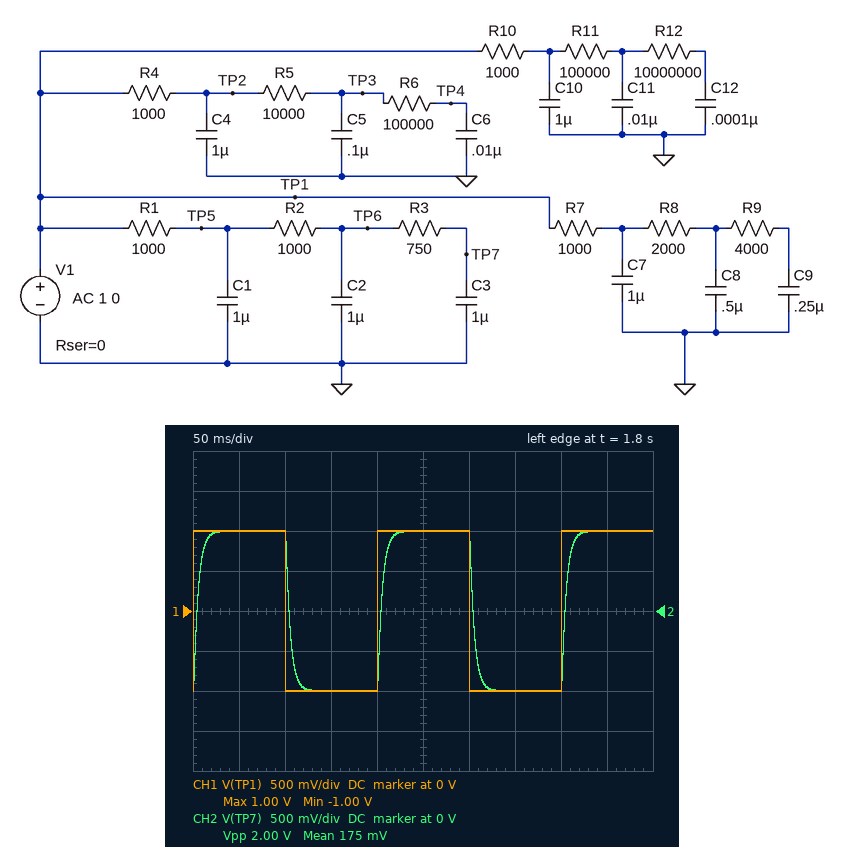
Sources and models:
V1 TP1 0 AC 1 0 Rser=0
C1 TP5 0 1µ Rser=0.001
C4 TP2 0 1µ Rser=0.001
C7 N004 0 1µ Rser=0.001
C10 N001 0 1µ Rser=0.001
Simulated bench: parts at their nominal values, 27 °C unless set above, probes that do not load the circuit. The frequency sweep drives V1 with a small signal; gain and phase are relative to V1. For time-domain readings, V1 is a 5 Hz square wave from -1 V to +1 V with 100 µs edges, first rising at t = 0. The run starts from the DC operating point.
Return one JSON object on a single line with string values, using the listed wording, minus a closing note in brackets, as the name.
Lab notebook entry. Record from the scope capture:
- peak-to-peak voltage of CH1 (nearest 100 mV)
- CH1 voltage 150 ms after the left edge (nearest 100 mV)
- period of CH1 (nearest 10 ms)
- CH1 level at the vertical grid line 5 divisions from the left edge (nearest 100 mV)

{"peak-to-peak voltage of CH1": "2.0 V", "CH1 voltage 150 ms after the left edge": "-1.0 V", "period of CH1": "200 ms", "CH1 level at the vertical grid line 5 divisions from the left edge": "1.0 V"}
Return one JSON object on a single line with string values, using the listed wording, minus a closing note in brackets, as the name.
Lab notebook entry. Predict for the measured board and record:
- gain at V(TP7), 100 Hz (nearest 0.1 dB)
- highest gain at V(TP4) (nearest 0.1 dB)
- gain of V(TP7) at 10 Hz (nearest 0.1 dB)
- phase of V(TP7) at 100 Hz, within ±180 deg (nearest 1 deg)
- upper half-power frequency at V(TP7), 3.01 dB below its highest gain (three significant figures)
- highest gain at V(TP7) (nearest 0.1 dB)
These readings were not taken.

{"gain at V(TP7), 100 Hz": "-10.9 dB", "highest gain at V(TP4)": "0 dB", "gain of V(TP7) at 10 Hz": "-0.4 dB", "phase of V(TP7) at 100 Hz, within ±180 deg": "-101 deg", "upper half-power frequency at V(TP7), 3.01 dB below its highest gain": "31.9 Hz", "highest gain at V(TP7)": "0 dB"}
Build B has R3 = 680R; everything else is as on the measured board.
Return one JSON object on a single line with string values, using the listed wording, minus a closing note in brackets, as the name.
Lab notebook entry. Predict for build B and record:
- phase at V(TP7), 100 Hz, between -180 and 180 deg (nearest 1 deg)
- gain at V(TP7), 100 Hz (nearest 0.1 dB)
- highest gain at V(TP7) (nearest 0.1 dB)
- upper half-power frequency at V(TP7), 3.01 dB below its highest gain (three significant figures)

{"phase at V(TP7), 100 Hz, between -180 and 180 deg": "-100 deg", "gain at V(TP7), 100 Hz": "-10.8 dB", "highest gain at V(TP7)": "0 dB", "upper half-power frequency at V(TP7), 3.01 dB below its highest gain": "32.1 Hz"}
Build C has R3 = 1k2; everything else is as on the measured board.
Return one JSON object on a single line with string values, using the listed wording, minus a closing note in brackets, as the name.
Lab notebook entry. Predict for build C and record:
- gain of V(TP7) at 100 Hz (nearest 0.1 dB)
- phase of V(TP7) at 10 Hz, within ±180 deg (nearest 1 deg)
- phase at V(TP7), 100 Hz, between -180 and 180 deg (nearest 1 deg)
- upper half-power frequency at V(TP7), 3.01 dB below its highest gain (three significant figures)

{"gain of V(TP7) at 100 Hz": "-11.6 dB", "phase of V(TP7) at 10 Hz, within ±180 deg": "-22 deg", "phase at V(TP7), 100 Hz, between -180 and 180 deg": "-109 deg", "upper half-power frequency at V(TP7), 3.01 dB below its highest gain": "30.2 Hz"}
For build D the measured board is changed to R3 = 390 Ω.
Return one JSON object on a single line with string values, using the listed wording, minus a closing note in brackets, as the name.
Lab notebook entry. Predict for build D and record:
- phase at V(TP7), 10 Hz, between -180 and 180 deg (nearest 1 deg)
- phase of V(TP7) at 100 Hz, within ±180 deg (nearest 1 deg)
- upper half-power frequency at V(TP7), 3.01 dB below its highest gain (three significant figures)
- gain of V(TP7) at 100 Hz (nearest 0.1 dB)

{"phase at V(TP7), 10 Hz, between -180 and 180 deg": "-19 deg", "phase of V(TP7) at 100 Hz, within ±180 deg": "-94 deg", "upper half-power frequency at V(TP7), 3.01 dB below its highest gain": "33.2 Hz", "gain of V(TP7) at 100 Hz": "-10.4 dB"}
